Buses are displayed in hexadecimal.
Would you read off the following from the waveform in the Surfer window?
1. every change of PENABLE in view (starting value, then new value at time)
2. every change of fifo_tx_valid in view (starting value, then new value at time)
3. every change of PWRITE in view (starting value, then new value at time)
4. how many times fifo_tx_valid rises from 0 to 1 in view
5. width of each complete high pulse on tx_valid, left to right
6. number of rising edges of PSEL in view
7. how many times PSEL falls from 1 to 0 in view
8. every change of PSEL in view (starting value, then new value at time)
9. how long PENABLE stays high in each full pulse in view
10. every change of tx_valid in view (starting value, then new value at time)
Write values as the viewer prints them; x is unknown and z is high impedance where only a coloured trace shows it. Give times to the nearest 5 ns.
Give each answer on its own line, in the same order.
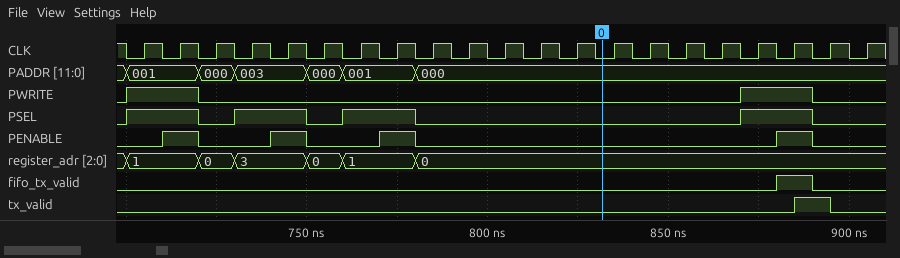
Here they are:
0, 1 at 710 ns, 0 at 720 ns, 1 at 740 ns, 0 at 750 ns, 1 at 770 ns, 0 at 780 ns, 1 at 880 ns, 0 at 890 ns
0, 1 at 880 ns, 0 at 890 ns
0, 1 at 700 ns, 0 at 720 ns, 1 at 870 ns, 0 at 890 ns
1
10 ns
4
4
0, 1 at 700 ns, 0 at 720 ns, 1 at 730 ns, 0 at 750 ns, 1 at 760 ns, 0 at 780 ns, 1 at 870 ns, 0 at 890 ns
10 ns, 10 ns, 10 ns, 10 ns
0, 1 at 885 ns, 0 at 895 ns
